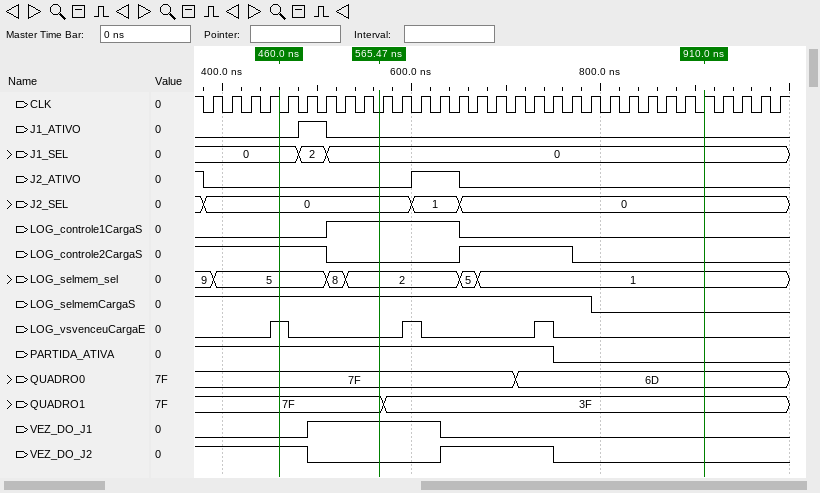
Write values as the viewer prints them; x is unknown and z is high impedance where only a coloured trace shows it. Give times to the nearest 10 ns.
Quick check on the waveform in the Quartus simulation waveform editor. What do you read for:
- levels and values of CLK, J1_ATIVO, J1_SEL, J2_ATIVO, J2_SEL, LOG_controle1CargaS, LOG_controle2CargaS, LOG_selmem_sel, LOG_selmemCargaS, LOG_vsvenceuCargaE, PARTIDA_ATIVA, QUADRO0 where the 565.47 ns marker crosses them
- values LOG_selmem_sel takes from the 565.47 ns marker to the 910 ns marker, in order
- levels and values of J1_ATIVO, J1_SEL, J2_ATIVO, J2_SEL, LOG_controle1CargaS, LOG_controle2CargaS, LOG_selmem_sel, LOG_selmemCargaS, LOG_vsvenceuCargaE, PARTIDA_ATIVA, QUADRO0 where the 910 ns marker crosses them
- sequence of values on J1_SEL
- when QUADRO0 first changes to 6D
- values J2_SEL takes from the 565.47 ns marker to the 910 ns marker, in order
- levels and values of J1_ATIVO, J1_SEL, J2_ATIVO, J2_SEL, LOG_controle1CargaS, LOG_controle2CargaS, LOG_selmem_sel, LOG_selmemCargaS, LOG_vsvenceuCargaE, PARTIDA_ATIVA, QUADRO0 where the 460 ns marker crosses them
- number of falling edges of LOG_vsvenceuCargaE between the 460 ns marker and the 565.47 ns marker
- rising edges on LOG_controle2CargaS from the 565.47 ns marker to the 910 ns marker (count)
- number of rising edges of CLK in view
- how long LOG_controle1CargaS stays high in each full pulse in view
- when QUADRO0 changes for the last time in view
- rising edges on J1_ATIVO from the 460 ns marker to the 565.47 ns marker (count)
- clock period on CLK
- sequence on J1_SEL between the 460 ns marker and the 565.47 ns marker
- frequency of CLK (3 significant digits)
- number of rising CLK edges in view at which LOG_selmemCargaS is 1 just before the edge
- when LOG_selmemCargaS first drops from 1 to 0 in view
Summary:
CLK=0, J1_ATIVO=0, J1_SEL=0, J2_ATIVO=0, J2_SEL=0, LOG_controle1CargaS=1, LOG_controle2CargaS=0, LOG_selmem_sel=2, LOG_selmemCargaS=1, LOG_vsvenceuCargaE=0, PARTIDA_ATIVA=1, QUADRO0=7F
2, 5, 1
J1_ATIVO=0, J1_SEL=0, J2_ATIVO=0, J2_SEL=0, LOG_controle1CargaS=0, LOG_controle2CargaS=0, LOG_selmem_sel=1, LOG_selmemCargaS=0, LOG_vsvenceuCargaE=0, PARTIDA_ATIVA=0, QUADRO0=6D
0, 2, 0
710 ns
0, 1, 0
J1_ATIVO=0, J1_SEL=0, J2_ATIVO=0, J2_SEL=0, LOG_controle1CargaS=0, LOG_controle2CargaS=1, LOG_selmem_sel=5, LOG_selmemCargaS=1, LOG_vsvenceuCargaE=1, PARTIDA_ATIVA=1, QUADRO0=7F
1
1
31
140 ns
710 ns
1
20 ns
0, 2, 0
50.0 MHz
21
790 ns
